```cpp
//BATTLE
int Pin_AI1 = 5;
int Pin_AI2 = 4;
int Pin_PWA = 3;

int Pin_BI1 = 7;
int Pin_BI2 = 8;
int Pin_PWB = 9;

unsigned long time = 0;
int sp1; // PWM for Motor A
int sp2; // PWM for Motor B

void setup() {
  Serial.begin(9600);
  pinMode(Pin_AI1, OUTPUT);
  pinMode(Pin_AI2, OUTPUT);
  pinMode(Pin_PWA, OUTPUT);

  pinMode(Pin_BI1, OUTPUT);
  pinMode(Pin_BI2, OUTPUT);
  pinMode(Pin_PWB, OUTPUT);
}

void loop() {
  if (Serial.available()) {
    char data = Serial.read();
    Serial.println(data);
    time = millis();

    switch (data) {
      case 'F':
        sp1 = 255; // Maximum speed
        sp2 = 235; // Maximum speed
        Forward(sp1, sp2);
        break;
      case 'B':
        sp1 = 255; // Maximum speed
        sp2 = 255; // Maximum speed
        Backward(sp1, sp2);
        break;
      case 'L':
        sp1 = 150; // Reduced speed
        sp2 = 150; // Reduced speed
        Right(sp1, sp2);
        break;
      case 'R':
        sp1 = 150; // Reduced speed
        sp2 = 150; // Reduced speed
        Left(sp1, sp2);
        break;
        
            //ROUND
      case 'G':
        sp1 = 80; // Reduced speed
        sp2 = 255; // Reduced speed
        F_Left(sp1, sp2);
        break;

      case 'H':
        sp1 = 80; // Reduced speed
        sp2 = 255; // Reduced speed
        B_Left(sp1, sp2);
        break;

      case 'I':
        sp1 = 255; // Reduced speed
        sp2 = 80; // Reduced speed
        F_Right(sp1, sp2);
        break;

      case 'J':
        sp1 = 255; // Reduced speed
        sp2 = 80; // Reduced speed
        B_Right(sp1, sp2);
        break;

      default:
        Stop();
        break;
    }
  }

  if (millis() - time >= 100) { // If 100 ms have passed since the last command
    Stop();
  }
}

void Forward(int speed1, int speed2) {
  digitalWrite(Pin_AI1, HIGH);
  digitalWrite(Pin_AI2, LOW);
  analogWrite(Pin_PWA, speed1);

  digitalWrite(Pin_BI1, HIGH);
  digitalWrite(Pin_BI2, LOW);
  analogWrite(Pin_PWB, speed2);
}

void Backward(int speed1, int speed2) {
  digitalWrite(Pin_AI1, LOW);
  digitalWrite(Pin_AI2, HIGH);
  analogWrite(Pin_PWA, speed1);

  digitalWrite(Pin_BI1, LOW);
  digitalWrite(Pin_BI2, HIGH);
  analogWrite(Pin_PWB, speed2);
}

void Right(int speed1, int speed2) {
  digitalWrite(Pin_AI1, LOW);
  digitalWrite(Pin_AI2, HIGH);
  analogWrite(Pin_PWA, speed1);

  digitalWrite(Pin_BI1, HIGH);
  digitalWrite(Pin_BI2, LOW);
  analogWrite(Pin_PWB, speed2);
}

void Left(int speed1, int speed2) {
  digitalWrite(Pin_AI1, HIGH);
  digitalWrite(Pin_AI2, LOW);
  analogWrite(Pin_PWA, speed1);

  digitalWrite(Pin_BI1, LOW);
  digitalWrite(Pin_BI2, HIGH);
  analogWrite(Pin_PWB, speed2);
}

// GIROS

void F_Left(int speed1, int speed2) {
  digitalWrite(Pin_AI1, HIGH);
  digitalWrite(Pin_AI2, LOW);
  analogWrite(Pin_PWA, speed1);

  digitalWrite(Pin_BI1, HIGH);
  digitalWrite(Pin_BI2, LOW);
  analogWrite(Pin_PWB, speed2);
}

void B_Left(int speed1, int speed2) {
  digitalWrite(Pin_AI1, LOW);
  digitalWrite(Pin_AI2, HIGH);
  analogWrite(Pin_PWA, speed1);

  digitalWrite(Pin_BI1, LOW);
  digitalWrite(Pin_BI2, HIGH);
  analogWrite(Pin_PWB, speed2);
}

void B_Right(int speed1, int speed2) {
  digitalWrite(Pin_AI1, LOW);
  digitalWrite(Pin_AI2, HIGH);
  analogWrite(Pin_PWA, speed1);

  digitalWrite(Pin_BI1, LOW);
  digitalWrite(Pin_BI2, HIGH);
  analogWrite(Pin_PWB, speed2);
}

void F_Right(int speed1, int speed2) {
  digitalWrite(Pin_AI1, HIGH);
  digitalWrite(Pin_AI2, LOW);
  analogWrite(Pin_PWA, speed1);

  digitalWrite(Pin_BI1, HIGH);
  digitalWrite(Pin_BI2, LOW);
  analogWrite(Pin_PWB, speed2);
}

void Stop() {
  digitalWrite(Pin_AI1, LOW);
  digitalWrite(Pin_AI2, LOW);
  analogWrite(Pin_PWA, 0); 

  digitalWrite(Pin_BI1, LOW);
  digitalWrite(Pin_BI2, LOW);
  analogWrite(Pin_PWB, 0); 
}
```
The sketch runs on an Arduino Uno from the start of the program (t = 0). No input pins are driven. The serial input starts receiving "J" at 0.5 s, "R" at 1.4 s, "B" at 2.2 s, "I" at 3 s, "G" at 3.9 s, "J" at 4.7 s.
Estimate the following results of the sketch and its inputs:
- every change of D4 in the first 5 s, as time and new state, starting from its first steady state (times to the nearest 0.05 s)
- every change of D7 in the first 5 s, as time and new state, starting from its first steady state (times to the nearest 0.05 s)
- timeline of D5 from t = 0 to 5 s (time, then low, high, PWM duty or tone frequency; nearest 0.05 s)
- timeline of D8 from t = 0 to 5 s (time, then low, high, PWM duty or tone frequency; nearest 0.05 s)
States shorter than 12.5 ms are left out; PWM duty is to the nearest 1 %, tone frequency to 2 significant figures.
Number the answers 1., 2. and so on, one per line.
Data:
1. 0 s low; 0.5 s high; 0.6 s low; 2.2 s high; 2.3 s low; 4.7 s high; 4.8 s low
2. 0 s low; 3 s high; 3.1 s low; 3.9 s high; 4 s low
3. 0 s low; 1.4 s high; 1.5 s low; 3 s high; 3.1 s low; 3.9 s high; 4 s low
4. 0 s low; 0.5 s high; 0.6 s low; 1.4 s high; 1.5 s low; 2.2 s high; 2.3 s low; 4.7 s high; 4.8 s low
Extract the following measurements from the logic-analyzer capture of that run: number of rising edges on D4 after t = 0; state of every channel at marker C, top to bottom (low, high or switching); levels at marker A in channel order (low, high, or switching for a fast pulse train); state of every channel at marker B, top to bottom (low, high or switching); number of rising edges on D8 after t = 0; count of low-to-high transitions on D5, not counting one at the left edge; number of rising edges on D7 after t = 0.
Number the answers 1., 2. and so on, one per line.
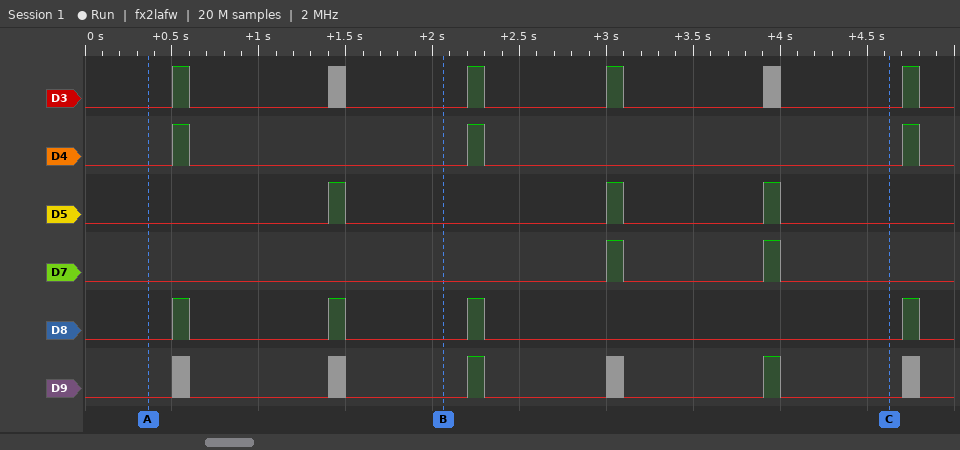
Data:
1. 3
2. D3 low, D4 low, D5 low, D7 low, D8 low, D9 low
3. D3 low, D4 low, D5 low, D7 low, D8 low, D9 low
4. D3 low, D4 low, D5 low, D7 low, D8 low, D9 low
5. 4
6. 3
7. 2
